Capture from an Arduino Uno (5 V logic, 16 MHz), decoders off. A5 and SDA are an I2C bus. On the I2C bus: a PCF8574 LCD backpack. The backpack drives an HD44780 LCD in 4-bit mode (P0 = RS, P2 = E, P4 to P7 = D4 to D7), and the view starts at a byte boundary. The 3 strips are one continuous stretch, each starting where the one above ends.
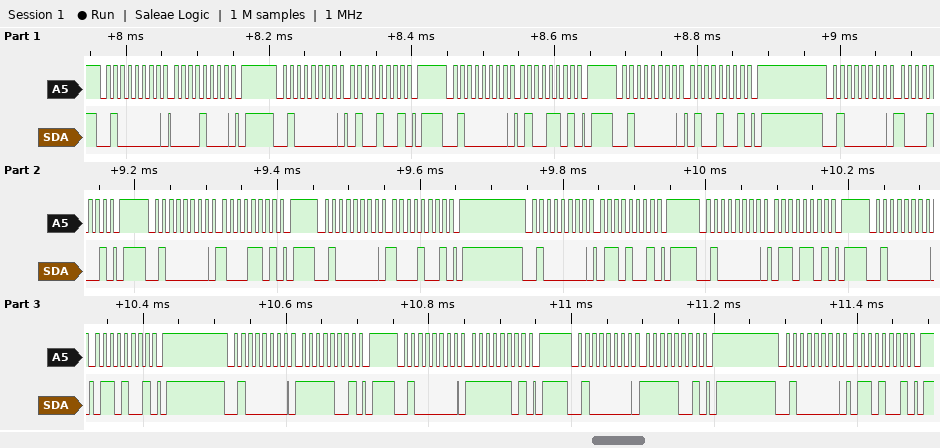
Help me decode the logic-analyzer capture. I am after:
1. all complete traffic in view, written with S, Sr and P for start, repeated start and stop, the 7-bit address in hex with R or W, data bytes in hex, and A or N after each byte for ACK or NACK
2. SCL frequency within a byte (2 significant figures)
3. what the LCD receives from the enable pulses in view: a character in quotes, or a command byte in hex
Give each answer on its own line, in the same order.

S 20W A 08 A P S 20W A 49 A P S 20W A 4D A P S 20W A 49 A P S 20W A 89 A P S 20W A 8D A P S 20W A 89 A P S 20W A 69 A P S 20W A 6D A P S 20W A 69 A P S 20W A F9 A P S 20W A FD A P S 20W A F9 A P S 20W A 69 A P
100 kHz
'H' 'o'
